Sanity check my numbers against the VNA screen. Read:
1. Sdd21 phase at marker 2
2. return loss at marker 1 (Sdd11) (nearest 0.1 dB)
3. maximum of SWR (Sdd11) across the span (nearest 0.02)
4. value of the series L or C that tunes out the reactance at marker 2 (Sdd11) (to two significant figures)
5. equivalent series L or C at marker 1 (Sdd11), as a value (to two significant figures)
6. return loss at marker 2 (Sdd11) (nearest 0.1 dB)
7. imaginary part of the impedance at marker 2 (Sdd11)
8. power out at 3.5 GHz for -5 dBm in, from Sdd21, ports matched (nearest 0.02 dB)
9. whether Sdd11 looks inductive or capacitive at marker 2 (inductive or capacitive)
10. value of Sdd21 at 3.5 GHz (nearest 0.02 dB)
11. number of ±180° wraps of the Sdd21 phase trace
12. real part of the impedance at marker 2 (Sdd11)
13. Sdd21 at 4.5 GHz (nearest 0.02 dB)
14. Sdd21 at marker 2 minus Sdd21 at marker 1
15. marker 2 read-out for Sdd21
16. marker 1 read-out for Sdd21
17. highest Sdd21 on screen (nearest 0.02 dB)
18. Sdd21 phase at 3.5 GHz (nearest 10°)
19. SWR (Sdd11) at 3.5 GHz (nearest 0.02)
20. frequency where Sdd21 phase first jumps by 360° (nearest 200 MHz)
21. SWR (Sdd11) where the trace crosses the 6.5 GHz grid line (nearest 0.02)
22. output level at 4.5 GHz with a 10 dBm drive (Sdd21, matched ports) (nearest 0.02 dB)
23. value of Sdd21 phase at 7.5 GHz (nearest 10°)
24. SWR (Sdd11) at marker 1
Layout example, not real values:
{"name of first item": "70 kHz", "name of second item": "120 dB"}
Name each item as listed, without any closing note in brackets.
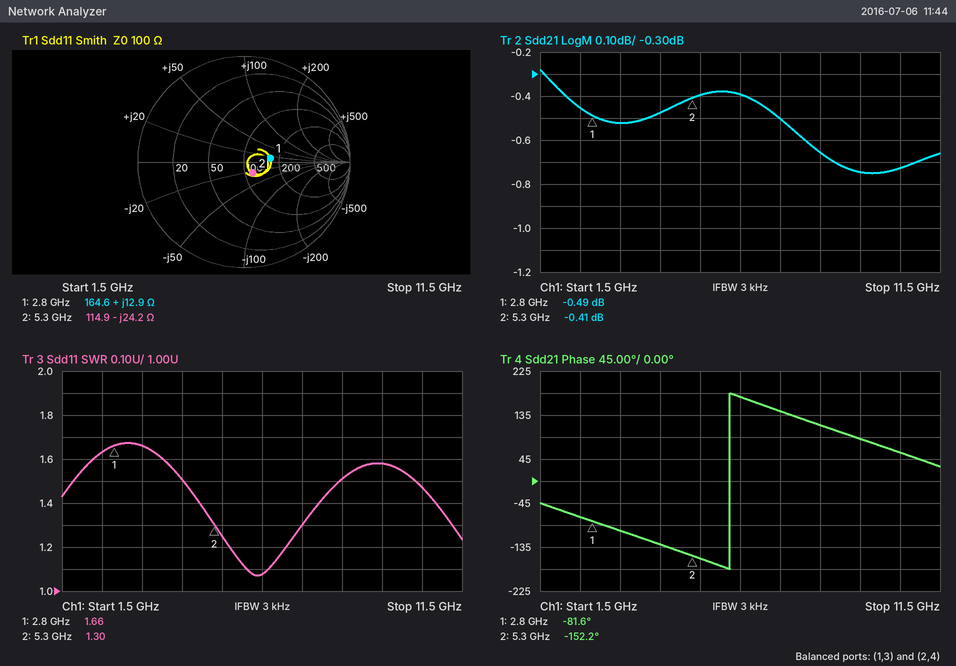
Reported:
{"Sdd21 phase at marker 2": "-152.2°", "return loss at marker 1 (Sdd11)": "12.1 dB", "maximum of SWR (Sdd11) across the span": "1.68", "value of the series L or C that tunes out the reactance at marker 2 (Sdd11)": "730 pH", "equivalent series L or C at marker 1 (Sdd11), as a value": "730 pH", "return loss at marker 2 (Sdd11)": "17.6 dB", "imaginary part of the impedance at marker 2": "-24.2 Ω", "power out at 3.5 GHz for -5 dBm in, from Sdd21, ports matched": "-5.52 dBm", "whether Sdd11 looks inductive or capacitive at marker 2": "capacitive", "value of Sdd21 at 3.5 GHz": "-0.52 dB", "number of ±180° wraps of the Sdd21 phase trace": "1", "real part of the impedance at marker 2": "114.9 Ω", "Sdd21 at 4.5 GHz": "-0.48 dB", "Sdd21 at marker 2 minus Sdd21 at marker 1": "0.08 dB", "marker 2 read-out for Sdd21": "-0.41 dB", "marker 1 read-out for Sdd21": "-0.49 dB", "highest Sdd21 on screen": "-0.28 dB", "Sdd21 phase at 3.5 GHz": "-100°", "SWR (Sdd11) at 3.5 GHz": "1.66", "frequency where Sdd21 phase first jumps by 360°": "6.2 GHz", "SWR (Sdd11) where the trace crosses the 6.5 GHz grid line": "1.08", "output level at 4.5 GHz with a 10 dBm drive (Sdd21, matched ports)": "9.52 dBm", "value of Sdd21 phase at 7.5 GHz": "140°", "SWR (Sdd11) at marker 1": "1.66"}
